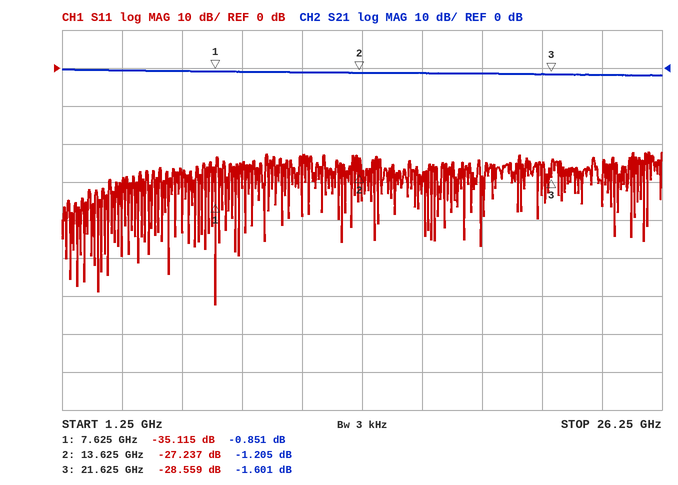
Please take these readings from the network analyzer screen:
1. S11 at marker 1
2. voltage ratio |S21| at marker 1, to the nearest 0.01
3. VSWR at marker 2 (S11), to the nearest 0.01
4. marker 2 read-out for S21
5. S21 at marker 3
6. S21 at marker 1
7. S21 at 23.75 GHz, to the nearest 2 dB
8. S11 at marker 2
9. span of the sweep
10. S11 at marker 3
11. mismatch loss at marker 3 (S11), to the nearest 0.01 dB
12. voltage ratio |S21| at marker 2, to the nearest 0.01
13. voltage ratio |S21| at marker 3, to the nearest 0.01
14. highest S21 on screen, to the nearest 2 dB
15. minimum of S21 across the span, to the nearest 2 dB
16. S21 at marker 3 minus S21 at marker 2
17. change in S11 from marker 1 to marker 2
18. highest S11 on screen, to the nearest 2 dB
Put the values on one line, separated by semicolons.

-35.115 dB; 0.91; 1.09; -1.205 dB; -1.601 dB; -0.851 dB; -2 dB; -27.237 dB; 25 GHz; -28.559 dB; 0.01 dB; 0.87; 0.83; 0 dB; -2 dB; -0.396 dB; 7.878 dB; -22 dB
